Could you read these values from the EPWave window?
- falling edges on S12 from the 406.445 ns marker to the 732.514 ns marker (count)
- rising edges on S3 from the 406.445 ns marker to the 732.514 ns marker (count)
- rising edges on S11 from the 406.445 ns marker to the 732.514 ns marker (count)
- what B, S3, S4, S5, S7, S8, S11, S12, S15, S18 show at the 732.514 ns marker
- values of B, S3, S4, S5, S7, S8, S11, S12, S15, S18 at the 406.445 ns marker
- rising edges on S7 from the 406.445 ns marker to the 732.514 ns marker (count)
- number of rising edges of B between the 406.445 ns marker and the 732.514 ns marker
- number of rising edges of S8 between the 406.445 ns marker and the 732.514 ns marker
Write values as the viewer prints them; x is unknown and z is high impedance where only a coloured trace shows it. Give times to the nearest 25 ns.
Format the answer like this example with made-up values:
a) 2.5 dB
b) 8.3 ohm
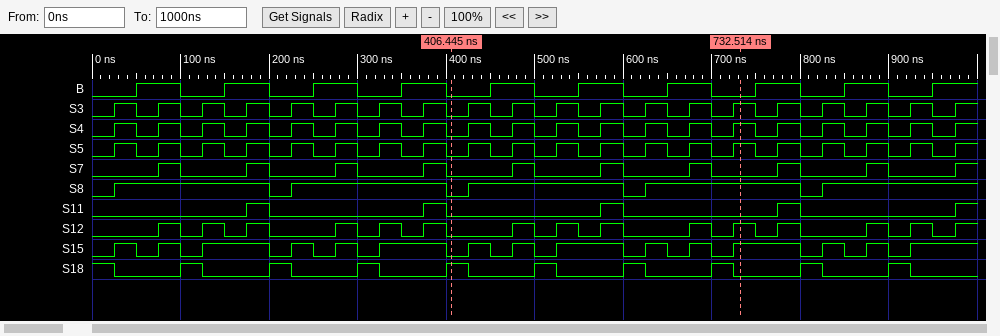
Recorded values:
a) 4
b) 7
c) 1
d) B=0, S3=1, S4=1, S5=1, S7=0, S8=1, S11=0, S12=1, S15=1, S18=0
e) B=0, S3=0, S4=0, S5=0, S7=0, S8=0, S11=0, S12=0, S15=0, S18=1
f) 3
g) 3
h) 2
